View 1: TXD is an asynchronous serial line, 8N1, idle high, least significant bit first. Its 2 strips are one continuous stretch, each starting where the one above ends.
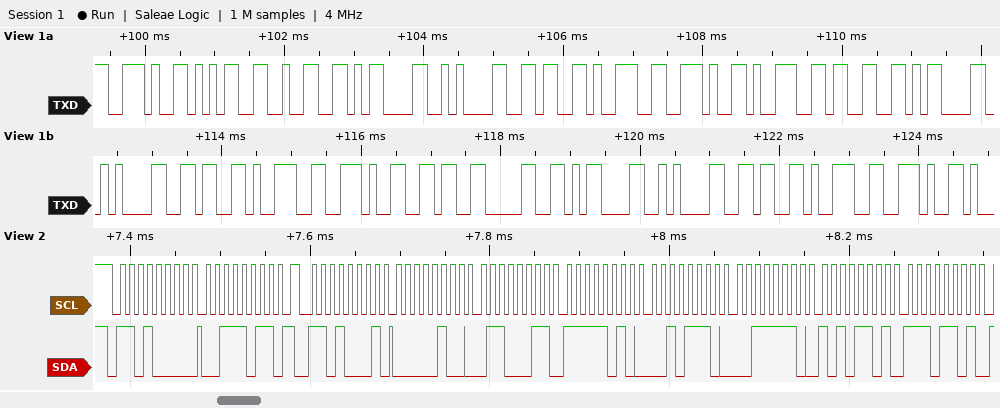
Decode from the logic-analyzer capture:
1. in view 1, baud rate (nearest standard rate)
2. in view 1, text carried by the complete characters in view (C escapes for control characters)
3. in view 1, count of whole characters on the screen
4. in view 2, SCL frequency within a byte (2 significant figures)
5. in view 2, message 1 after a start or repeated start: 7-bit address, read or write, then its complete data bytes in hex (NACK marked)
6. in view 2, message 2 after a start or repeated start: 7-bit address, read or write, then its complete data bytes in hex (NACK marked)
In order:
9600 baud
".52\r\n69.93\r\n69.60\r\n69."
22
100 kHz
0x68 write: 3B
0x68 read: 04 63 FA 2E 3E AD ED
